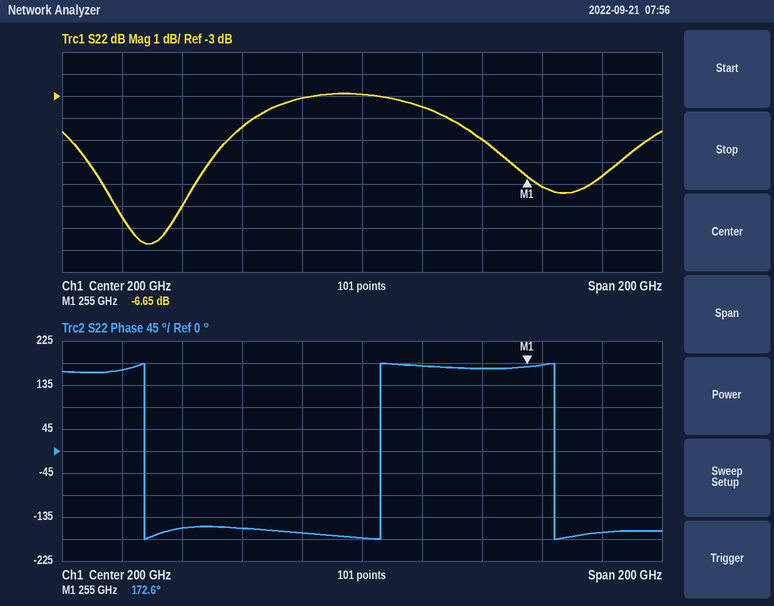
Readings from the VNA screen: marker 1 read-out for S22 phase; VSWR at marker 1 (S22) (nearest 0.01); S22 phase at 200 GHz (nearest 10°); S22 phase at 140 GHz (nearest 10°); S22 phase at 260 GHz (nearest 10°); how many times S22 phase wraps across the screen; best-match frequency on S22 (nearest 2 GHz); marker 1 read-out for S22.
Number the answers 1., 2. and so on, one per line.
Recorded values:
1. 172.6°
2. 2.74
3. -180°
4. -160°
5. 180°
6. 3
7. 128 GHz
8. -6.65 dB
